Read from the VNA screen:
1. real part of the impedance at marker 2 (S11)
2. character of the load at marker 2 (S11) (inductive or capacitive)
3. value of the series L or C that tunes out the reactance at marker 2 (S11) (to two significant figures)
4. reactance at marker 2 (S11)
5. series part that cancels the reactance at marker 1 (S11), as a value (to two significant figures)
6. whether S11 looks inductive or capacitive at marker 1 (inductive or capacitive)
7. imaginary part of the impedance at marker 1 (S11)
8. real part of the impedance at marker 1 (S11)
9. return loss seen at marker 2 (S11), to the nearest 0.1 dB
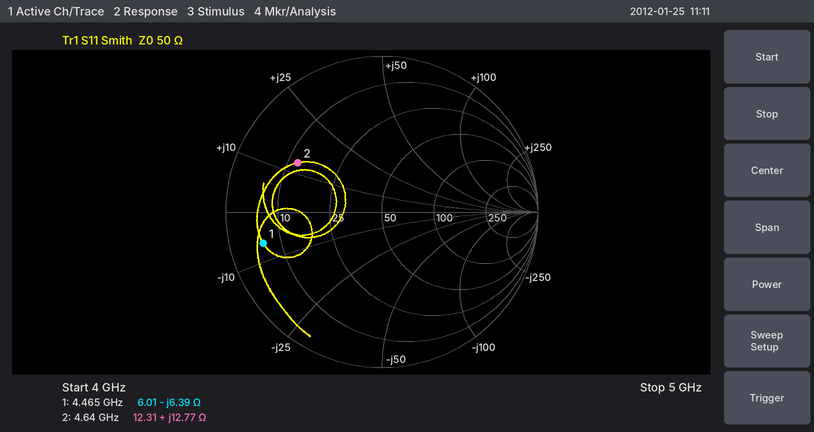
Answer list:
12.31 Ω
inductive
2.7 pF
+12.77 Ω
230 pH
capacitive
-6.39 Ω
6.01 Ω
4.1 dB
